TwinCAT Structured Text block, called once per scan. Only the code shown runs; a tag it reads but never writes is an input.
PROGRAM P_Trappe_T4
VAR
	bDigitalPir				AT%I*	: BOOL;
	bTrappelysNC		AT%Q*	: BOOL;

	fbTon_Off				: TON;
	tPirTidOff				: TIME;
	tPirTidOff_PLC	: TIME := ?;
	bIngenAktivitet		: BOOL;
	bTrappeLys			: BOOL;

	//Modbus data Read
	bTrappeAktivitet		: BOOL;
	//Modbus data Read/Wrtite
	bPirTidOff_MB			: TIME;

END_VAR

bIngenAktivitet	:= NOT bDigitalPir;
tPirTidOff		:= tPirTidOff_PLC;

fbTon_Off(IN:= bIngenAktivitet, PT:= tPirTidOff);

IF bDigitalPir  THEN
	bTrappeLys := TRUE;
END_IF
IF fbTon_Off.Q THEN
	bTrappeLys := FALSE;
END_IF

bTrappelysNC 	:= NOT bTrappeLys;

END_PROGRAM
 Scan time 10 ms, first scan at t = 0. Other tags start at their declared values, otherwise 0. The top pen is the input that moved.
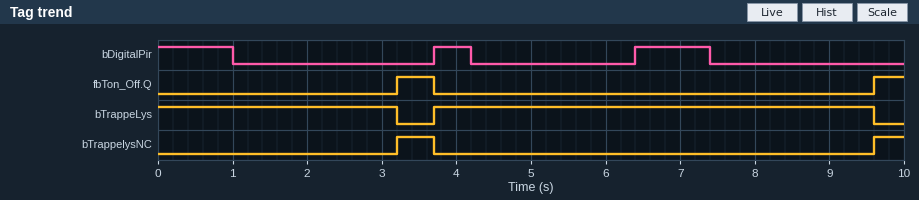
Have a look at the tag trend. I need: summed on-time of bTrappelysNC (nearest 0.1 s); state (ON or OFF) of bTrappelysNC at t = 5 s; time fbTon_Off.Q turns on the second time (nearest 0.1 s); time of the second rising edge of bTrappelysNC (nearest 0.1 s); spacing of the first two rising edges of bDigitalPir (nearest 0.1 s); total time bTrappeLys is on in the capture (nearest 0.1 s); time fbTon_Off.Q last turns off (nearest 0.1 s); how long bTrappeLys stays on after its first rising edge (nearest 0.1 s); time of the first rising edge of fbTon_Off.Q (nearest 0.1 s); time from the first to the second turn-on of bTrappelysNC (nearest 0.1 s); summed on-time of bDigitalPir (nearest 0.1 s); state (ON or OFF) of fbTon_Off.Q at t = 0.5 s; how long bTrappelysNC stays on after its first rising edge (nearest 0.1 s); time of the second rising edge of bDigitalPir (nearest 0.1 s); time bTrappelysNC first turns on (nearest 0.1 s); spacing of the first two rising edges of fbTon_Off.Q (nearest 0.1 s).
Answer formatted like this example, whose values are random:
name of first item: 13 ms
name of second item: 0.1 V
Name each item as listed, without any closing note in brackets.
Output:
summed on-time of bTrappelysNC: 0.9 s
state (ON or OFF) of bTrappelysNC at t = 5 s: OFF
time fbTon_Off.Q turns on the second time: 9.6 s
time of the second rising edge of bTrappelysNC: 9.6 s
spacing of the first two rising edges of bDigitalPir: 2.7 s
total time bTrappeLys is on in the capture: 9.1 s
time fbTon_Off.Q last turns off: 3.7 s
how long bTrappeLys stays on after its first rising edge: 5.9 s
time of the first rising edge of fbTon_Off.Q: 3.2 s
time from the first to the second turn-on of bTrappelysNC: 6.4 s
summed on-time of bDigitalPir: 2.5 s
state (ON or OFF) of fbTon_Off.Q at t = 0.5 s: OFF
how long bTrappelysNC stays on after its first rising edge: 0.5 s
time of the second rising edge of bDigitalPir: 6.4 s
time bTrappelysNC first turns on: 3.2 s
spacing of the first two rising edges of fbTon_Off.Q: 6.4 s
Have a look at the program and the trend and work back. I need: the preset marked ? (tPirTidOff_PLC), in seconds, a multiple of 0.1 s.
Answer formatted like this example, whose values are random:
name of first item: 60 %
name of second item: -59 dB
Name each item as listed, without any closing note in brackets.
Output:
the preset marked ? (tPirTidOff_PLC), in seconds, a multiple of 0.1 s: 2.2 s
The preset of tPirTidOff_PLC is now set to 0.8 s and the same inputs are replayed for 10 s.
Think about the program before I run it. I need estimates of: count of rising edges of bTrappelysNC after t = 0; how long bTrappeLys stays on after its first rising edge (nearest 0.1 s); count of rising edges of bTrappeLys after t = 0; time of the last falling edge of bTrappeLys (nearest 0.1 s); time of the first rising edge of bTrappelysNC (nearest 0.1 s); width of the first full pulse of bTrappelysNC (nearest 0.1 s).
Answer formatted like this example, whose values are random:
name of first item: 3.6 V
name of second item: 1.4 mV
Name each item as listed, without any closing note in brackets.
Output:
count of rising edges of bTrappelysNC after t = 0: 3
how long bTrappeLys stays on after its first rising edge: 1.3 s
count of rising edges of bTrappeLys after t = 0: 2
time of the last falling edge of bTrappeLys: 8.2 s
time of the first rising edge of bTrappelysNC: 1.8 s
width of the first full pulse of bTrappelysNC: 1.9 s
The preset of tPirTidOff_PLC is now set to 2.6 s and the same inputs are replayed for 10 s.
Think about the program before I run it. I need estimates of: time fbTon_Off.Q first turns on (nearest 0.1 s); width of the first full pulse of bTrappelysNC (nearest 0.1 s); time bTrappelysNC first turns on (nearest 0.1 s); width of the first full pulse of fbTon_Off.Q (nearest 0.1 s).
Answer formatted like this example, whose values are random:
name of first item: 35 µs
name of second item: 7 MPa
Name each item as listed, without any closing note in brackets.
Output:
time fbTon_Off.Q first turns on: 3.6 s
width of the first full pulse of bTrappelysNC: 0.1 s
time bTrappelysNC first turns on: 3.6 s
width of the first full pulse of fbTon_Off.Q: 0.1 s
